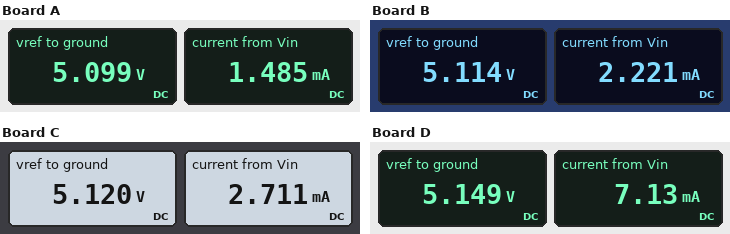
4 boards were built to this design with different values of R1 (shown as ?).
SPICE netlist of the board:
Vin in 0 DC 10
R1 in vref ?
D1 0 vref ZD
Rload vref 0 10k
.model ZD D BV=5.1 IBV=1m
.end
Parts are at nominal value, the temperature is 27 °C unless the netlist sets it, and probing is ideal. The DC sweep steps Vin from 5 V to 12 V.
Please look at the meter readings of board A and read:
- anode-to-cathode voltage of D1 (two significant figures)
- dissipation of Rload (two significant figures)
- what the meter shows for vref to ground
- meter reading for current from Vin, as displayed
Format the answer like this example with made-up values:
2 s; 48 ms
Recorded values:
-5.1 V; 2.6 mW; 5.099 V; 1.485 mA
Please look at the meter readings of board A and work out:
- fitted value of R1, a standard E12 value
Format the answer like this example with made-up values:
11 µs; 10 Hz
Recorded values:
3.3 kΩ
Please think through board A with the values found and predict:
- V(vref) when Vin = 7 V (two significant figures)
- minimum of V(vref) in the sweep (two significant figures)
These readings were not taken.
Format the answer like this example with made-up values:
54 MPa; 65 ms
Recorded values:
5.0 V; 3.8 V
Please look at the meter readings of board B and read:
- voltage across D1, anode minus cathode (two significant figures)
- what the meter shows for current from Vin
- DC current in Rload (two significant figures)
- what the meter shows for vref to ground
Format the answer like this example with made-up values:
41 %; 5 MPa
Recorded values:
-5.1 V; 2.221 mA; 510 µA; 5.114 V
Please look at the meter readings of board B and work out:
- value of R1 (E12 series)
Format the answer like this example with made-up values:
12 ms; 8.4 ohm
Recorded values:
2.2 kΩ
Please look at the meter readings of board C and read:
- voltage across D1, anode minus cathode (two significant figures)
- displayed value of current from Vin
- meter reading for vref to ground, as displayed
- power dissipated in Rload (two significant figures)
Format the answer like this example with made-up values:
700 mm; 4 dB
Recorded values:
-5.1 V; 2.711 mA; 5.120 V; 2.6 mW
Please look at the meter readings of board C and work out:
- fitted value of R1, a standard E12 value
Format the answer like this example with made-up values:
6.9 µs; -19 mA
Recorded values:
1.8 kΩ
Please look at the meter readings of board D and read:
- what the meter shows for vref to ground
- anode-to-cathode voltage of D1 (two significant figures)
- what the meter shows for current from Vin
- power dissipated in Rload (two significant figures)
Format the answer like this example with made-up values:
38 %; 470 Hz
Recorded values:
5.149 V; -5.1 V; 7.13 mA; 2.7 mW
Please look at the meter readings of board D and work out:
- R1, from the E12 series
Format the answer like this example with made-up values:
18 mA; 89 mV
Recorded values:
680 Ω
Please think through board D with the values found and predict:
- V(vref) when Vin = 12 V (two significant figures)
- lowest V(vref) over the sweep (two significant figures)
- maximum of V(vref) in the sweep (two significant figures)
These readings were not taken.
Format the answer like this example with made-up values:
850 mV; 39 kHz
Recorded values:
5.2 V; 4.7 V; 5.2 V
